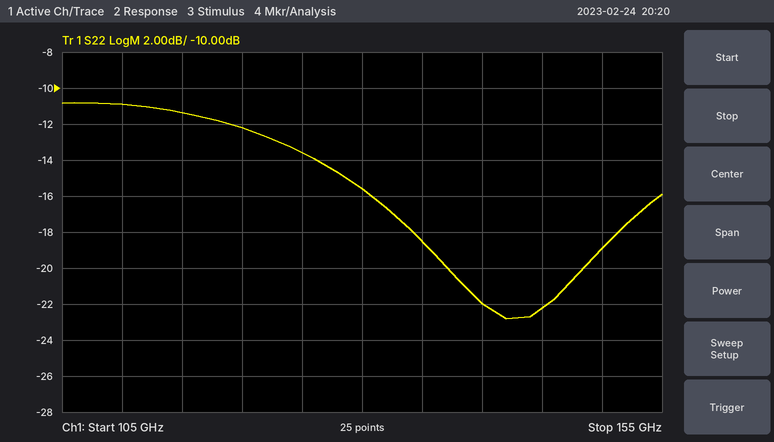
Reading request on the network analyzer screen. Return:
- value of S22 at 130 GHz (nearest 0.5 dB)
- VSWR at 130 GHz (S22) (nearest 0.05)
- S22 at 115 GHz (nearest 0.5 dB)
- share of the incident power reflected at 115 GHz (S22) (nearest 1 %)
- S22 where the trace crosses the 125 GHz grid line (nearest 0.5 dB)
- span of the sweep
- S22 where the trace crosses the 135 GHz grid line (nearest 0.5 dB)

-15.5 dB
1.40
-11.5 dB
7 %
-13.5 dB
50 GHz
-18.5 dB
